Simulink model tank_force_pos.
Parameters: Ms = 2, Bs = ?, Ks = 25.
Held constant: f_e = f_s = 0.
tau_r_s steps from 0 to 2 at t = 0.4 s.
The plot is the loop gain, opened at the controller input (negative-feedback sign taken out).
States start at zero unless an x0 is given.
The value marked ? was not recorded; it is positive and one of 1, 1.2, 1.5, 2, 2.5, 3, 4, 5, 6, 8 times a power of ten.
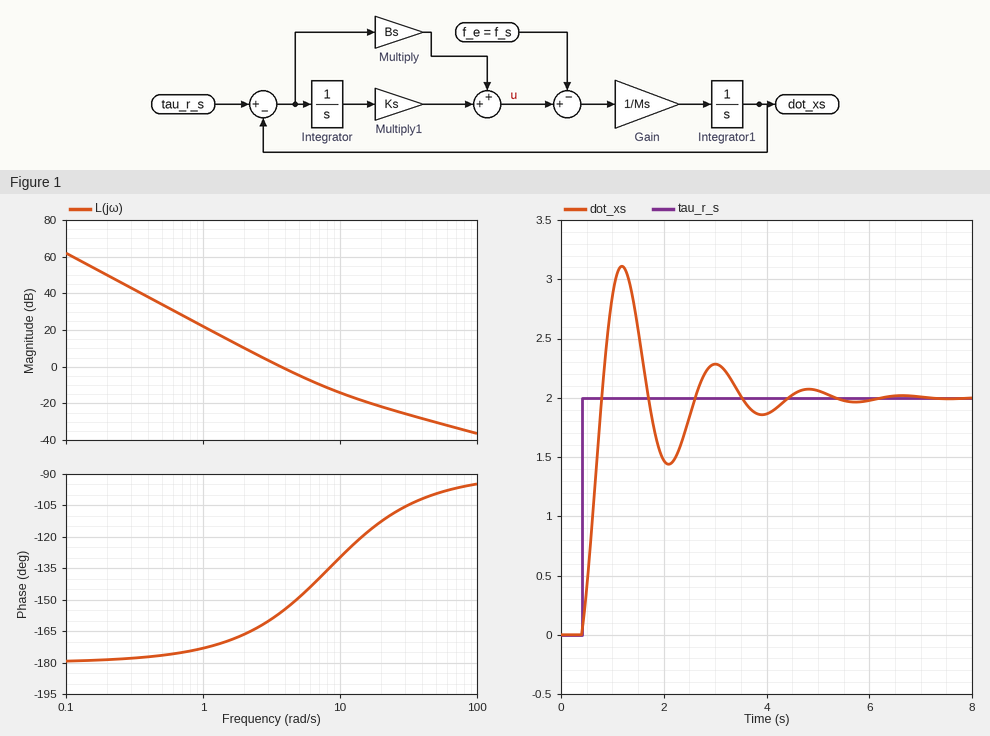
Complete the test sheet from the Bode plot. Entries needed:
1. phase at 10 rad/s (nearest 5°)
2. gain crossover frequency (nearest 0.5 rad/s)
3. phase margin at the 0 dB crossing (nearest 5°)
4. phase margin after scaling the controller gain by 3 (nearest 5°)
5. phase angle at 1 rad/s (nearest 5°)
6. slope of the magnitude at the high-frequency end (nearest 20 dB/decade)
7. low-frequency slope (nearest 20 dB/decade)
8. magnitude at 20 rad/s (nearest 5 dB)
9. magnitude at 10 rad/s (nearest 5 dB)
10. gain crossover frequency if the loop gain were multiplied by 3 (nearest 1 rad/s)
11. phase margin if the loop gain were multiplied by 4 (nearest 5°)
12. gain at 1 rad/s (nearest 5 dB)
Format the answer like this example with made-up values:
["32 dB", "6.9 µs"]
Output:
["-130°", "3.5 rad/s", "25°", "40°", "-175°", "-20 dB/decade", "-40 dB/decade", "-20 dB", "-15 dB", "7 rad/s", "45°", "20 dB"]
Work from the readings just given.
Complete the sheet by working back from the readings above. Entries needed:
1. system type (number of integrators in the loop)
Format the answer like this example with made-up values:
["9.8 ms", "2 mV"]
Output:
["2"]
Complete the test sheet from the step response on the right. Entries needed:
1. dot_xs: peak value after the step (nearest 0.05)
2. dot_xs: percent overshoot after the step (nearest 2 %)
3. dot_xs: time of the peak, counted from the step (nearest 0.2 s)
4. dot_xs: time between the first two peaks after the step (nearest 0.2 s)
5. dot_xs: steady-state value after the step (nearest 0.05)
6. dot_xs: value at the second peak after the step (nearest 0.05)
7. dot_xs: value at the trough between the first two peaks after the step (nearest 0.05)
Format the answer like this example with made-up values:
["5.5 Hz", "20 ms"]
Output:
["3.10", "56 %", "0.8 s", "1.8 s", "2.00", "2.30", "1.45"]
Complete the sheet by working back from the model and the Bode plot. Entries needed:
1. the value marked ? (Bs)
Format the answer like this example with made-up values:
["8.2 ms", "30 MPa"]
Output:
["3"]
